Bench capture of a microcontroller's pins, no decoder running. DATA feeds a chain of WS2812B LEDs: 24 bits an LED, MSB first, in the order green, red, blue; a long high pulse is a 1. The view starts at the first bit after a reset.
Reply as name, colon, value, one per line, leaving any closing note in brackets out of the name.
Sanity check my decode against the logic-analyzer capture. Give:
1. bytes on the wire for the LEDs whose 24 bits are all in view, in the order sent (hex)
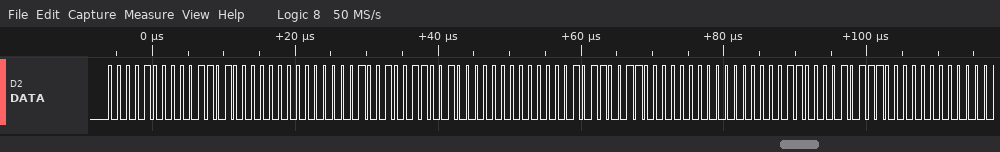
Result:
bytes on the wire for the LEDs whose 24 bits are all in view, in the order sent: 08 34 00 09 32 00 0B 30 00 0C 2E 00
